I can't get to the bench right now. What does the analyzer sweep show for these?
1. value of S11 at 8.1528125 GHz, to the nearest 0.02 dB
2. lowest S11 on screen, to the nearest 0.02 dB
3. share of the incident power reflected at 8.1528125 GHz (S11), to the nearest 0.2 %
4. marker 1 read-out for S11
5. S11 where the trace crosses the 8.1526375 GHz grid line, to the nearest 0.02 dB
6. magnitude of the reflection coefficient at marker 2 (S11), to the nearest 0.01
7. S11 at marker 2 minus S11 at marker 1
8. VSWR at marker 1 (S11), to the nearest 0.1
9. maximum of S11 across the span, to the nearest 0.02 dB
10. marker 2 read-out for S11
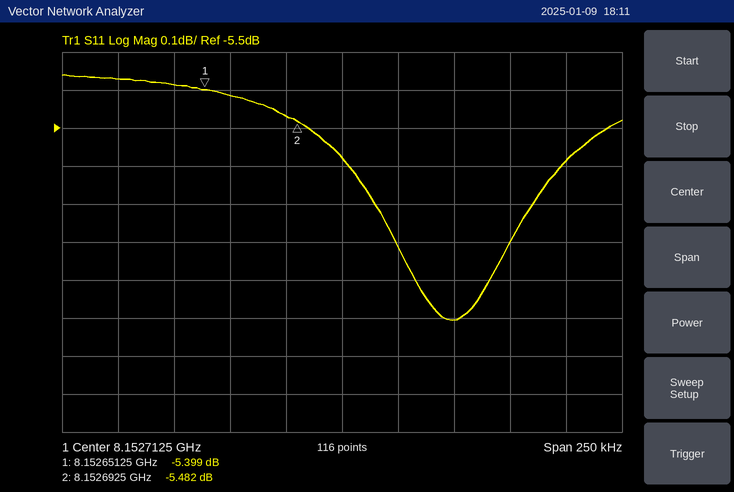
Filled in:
-5.58 dB
-6.00 dB
27.6 %
-5.399 dB
-5.38 dB
0.53
-0.083 dB
3.3
-5.36 dB
-5.482 dB
